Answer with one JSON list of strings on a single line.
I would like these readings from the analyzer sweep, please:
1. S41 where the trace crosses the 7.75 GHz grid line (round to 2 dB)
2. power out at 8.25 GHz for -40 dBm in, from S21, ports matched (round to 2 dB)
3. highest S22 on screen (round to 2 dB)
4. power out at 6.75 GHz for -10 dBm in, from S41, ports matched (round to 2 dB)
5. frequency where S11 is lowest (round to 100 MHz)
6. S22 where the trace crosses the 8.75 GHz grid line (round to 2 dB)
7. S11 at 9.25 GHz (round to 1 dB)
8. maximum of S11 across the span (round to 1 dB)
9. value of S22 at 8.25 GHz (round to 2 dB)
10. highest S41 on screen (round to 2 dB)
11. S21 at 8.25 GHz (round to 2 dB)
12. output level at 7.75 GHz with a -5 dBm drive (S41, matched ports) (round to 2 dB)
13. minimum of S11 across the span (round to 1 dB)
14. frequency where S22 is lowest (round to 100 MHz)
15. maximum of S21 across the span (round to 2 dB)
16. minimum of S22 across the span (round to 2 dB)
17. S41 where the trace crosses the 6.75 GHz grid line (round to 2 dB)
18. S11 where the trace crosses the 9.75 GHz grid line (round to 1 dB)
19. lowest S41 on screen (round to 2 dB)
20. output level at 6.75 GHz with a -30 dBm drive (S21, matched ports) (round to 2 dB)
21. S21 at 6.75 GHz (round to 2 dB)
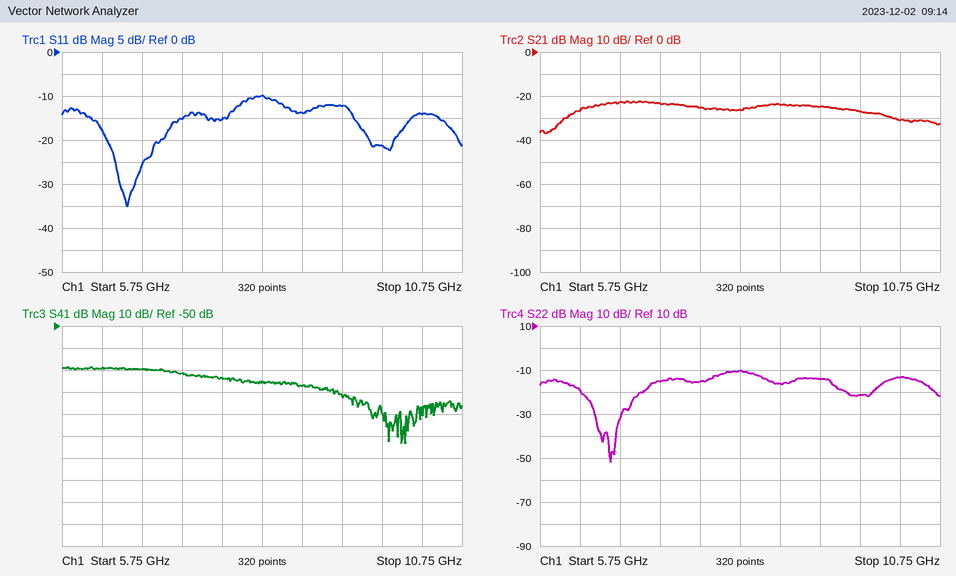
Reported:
["-74 dB", "-66 dBm", "-10 dB", "-80 dBm", "6.6 GHz", "-16 dB", "-12 dB", "-10 dB", "-10 dB", "-68 dB", "-26 dB", "-78 dBm", "-35 dB", "6.6 GHz", "-22 dB", "-52 dB", "-70 dB", "-21 dB", "-104 dB", "-52 dBm", "-22 dB"]
